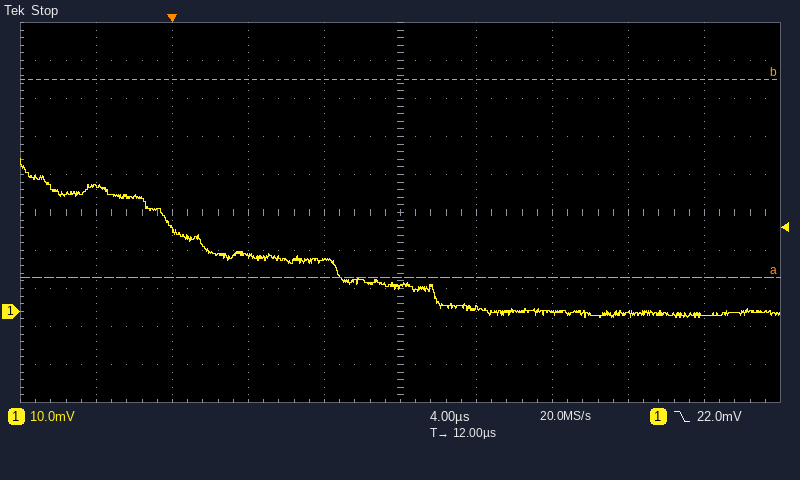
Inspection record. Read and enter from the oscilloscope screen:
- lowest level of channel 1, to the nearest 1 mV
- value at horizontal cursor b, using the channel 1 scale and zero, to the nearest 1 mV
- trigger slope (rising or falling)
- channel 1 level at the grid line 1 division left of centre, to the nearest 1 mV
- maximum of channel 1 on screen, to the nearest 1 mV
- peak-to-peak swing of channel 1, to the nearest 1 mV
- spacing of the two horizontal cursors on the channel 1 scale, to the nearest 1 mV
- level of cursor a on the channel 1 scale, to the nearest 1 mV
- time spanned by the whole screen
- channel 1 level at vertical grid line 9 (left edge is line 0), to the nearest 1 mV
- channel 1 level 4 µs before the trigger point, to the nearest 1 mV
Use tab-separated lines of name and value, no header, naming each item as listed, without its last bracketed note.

lowest level of channel 1, to the nearest 1 mV	-2 mV
value at horizontal cursor b, using the channel 1 scale and zero, to the nearest 1 mV	61 mV
trigger slope	falling
channel 1 level at the grid line 1 division left of centre, to the nearest 1 mV	14 mV
maximum of channel 1 on screen, to the nearest 1 mV	40 mV
peak-to-peak swing of channel 1, to the nearest 1 mV	42 mV
spacing of the two horizontal cursors on the channel 1 scale, to the nearest 1 mV	52 mV
level of cursor a on the channel 1 scale, to the nearest 1 mV	9 mV
time spanned by the whole screen	40 µs
channel 1 level at vertical grid line 9 (left edge is line 0), to the nearest 1 mV	-1 mV
channel 1 level 4 µs before the trigger point, to the nearest 1 mV	33 mV
